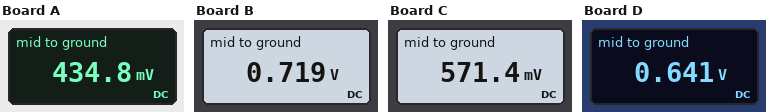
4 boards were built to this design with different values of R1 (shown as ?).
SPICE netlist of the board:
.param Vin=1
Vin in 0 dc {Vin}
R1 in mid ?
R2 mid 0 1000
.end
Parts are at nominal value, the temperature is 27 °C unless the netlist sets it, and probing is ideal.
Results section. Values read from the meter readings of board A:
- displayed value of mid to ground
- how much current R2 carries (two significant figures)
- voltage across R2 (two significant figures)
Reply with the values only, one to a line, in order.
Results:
434.8 mV
430 µA
430 mV
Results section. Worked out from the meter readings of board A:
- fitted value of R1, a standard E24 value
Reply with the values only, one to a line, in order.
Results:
1.3 kΩ
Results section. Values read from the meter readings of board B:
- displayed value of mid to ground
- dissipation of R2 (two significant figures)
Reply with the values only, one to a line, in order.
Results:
0.719 V
520 µW
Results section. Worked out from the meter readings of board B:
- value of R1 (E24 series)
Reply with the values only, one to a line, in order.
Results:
390 Ω
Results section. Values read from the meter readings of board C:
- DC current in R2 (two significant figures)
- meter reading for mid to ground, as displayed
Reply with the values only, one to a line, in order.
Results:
570 µA
571.4 mV
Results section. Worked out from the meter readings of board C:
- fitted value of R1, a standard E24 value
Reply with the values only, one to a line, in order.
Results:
750 Ω
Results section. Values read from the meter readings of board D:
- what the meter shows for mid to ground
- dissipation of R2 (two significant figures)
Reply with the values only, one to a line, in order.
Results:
0.641 V
410 µW
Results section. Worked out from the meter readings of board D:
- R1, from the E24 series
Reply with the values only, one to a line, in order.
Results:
560 Ω
